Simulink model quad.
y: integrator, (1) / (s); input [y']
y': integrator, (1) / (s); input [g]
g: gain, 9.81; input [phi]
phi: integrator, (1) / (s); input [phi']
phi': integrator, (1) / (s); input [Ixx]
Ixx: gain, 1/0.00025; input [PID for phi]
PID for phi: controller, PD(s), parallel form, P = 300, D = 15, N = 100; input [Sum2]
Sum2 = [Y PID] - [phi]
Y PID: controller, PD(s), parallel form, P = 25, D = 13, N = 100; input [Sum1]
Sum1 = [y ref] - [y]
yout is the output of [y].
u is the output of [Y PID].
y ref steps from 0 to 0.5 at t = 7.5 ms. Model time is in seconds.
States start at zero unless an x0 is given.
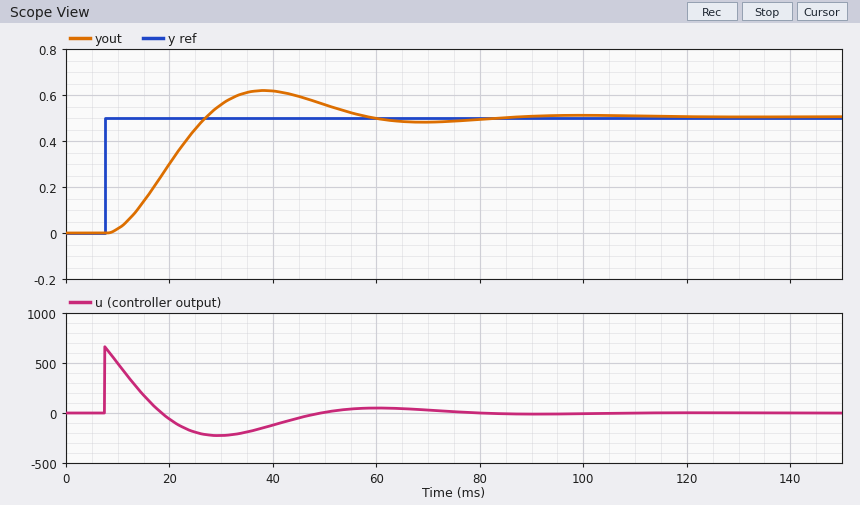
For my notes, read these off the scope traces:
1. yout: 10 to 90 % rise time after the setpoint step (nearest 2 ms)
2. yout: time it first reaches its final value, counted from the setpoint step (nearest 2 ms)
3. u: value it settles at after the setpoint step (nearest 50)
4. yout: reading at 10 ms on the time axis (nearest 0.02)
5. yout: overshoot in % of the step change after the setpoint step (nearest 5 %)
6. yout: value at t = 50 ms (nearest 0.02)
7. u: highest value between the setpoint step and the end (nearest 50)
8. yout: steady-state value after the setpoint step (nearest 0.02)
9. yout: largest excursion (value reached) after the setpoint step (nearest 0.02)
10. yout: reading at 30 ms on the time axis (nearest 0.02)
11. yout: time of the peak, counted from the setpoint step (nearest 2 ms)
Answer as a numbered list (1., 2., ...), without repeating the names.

1. 14 ms
2. 20 ms
3. 0
4. 0.02
5. 25 %
6. 0.56
7. 650
8. 0.50
9. 0.62
10. 0.56
11. 30 ms
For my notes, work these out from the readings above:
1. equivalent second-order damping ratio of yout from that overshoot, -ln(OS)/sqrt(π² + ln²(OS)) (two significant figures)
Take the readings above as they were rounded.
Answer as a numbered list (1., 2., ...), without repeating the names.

1. 0.40
